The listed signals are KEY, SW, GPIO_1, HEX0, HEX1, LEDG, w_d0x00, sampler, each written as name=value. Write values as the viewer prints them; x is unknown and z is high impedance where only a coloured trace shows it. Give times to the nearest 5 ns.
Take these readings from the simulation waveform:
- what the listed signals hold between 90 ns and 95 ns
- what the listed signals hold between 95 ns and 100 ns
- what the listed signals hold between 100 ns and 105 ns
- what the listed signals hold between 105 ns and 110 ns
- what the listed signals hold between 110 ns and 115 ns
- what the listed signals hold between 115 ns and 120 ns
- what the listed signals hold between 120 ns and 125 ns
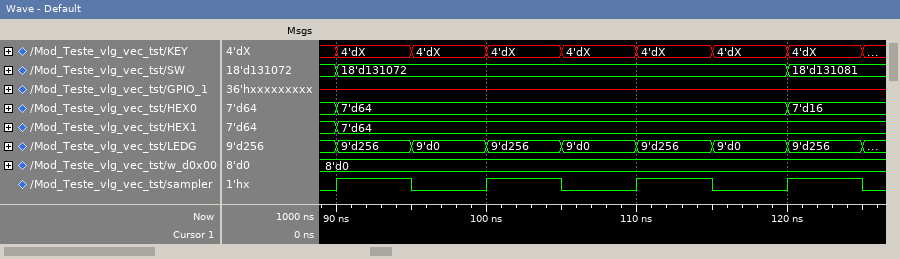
KEY=4'dX, SW=18'd131072, GPIO_1=x, HEX0=7'd64, HEX1=7'd64, LEDG=9'd256, w_d0x00=8'd0, sampler=1
KEY=4'dX, SW=18'd131072, GPIO_1=x, HEX0=7'd64, HEX1=7'd64, LEDG=9'd0, w_d0x00=8'd0, sampler=0
KEY=4'dX, SW=18'd131072, GPIO_1=x, HEX0=7'd64, HEX1=7'd64, LEDG=9'd256, w_d0x00=8'd0, sampler=1
KEY=4'dX, SW=18'd131072, GPIO_1=x, HEX0=7'd64, HEX1=7'd64, LEDG=9'd0, w_d0x00=8'd0, sampler=0
KEY=4'dX, SW=18'd131072, GPIO_1=x, HEX0=7'd64, HEX1=7'd64, LEDG=9'd256, w_d0x00=8'd0, sampler=1
KEY=4'dX, SW=18'd131072, GPIO_1=x, HEX0=7'd64, HEX1=7'd64, LEDG=9'd0, w_d0x00=8'd0, sampler=0
KEY=4'dX, SW=18'd131081, GPIO_1=x, HEX0=7'd16, HEX1=7'd64, LEDG=9'd256, w_d0x00=8'd0, sampler=1
